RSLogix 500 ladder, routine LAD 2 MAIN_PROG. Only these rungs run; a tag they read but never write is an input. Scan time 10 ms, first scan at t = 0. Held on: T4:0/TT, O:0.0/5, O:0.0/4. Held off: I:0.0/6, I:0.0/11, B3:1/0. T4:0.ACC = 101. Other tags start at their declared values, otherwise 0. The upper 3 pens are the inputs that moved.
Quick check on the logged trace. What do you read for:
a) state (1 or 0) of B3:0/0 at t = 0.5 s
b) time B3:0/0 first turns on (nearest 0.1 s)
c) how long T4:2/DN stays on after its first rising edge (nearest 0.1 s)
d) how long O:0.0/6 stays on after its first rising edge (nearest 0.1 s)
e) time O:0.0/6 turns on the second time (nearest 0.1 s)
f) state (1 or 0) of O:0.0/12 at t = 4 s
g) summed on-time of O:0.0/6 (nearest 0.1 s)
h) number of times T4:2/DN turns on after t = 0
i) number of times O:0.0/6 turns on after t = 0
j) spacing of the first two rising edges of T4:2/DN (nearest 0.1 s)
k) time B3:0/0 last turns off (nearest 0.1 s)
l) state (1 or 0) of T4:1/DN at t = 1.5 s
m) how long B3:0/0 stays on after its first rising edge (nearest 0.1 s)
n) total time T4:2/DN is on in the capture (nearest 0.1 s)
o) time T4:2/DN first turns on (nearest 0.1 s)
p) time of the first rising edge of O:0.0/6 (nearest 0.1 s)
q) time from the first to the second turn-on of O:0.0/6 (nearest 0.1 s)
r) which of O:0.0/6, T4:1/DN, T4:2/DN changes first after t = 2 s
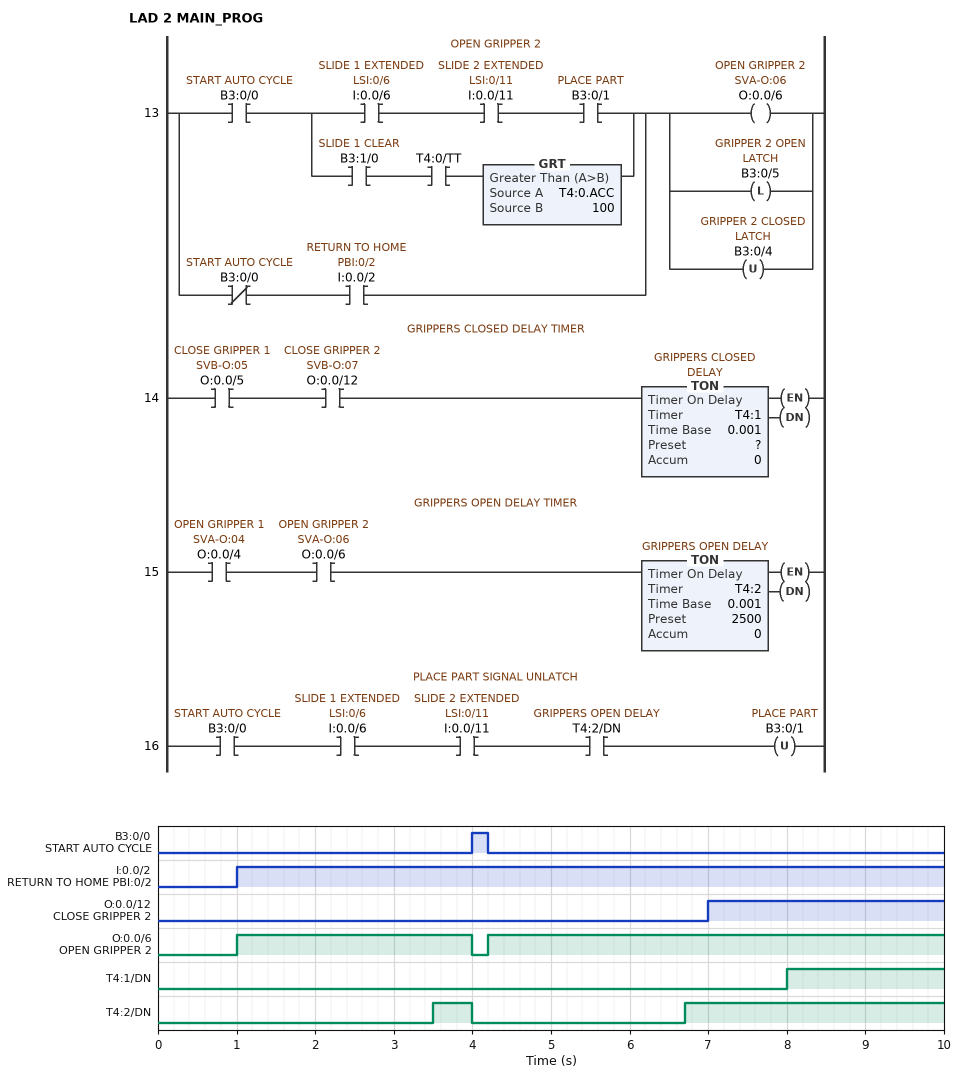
0
4.0 s
0.5 s
3.0 s
4.2 s
0
8.8 s
2
2
3.2 s
4.2 s
0
0.2 s
3.8 s
3.5 s
1.0 s
3.2 s
T4:2/DN
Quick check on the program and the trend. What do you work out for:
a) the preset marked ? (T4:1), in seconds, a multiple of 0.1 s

1.0 s
